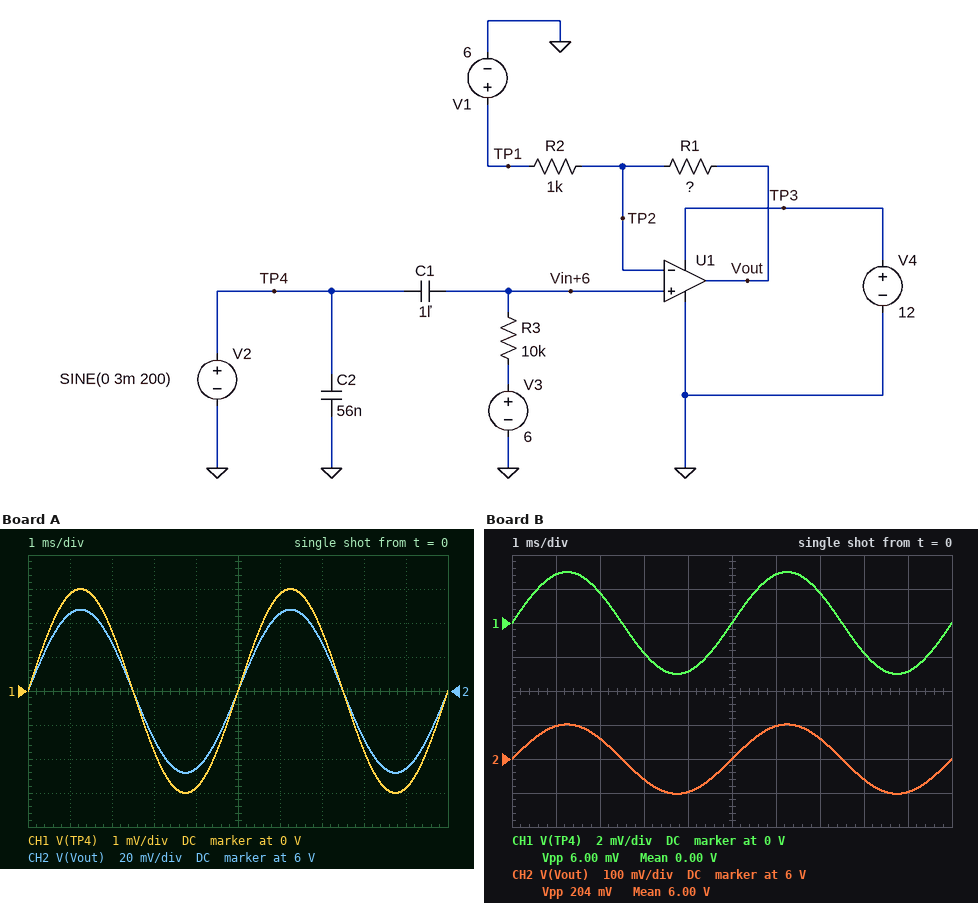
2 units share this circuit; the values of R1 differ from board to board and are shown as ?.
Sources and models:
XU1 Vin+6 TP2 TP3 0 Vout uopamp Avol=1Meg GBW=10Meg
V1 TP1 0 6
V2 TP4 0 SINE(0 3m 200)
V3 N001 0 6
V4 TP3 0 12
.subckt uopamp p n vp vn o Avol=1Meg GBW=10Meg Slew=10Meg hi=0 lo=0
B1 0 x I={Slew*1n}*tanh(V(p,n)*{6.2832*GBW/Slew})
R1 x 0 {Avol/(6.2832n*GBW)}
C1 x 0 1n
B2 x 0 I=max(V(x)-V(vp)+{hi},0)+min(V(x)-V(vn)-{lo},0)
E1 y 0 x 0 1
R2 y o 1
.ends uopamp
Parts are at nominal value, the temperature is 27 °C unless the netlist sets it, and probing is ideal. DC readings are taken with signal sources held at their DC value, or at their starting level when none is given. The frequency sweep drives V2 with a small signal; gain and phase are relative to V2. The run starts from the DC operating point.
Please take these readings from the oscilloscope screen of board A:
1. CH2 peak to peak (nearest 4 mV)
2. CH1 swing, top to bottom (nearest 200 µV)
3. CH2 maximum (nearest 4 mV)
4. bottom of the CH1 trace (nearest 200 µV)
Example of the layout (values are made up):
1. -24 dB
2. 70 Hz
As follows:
1. 96 mV
2. 6.0 mV
3. 6.048 V
4. -3.0 mV
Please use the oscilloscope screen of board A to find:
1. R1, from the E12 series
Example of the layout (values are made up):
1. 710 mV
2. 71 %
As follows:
1. 15 kΩ
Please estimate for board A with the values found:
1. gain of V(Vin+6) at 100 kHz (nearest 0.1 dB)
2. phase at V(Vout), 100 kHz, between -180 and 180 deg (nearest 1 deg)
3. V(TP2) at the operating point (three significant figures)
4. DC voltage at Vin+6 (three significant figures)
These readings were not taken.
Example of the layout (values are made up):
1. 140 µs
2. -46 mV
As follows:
1. 0 dB
2. -9 deg
3. 6.00 V
4. 6.00 V
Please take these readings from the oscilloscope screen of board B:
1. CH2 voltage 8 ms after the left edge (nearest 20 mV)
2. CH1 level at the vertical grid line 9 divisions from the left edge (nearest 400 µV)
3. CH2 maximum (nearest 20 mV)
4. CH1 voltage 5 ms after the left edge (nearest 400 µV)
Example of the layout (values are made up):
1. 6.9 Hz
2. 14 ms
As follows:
1. 5.94 V
2. -2.8 mV
3. 6.10 V
4. 0 V
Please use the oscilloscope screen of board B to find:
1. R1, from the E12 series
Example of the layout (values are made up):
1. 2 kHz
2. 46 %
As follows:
1. 33 kΩ
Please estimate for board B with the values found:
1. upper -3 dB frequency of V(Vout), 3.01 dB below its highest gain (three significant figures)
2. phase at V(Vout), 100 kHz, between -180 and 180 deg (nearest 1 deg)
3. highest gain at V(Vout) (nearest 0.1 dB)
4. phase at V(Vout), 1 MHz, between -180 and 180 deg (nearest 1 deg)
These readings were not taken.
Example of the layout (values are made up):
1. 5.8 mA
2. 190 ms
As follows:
1. 294 kHz
2. -19 deg
3. 30.6 dB
4. -74 deg
